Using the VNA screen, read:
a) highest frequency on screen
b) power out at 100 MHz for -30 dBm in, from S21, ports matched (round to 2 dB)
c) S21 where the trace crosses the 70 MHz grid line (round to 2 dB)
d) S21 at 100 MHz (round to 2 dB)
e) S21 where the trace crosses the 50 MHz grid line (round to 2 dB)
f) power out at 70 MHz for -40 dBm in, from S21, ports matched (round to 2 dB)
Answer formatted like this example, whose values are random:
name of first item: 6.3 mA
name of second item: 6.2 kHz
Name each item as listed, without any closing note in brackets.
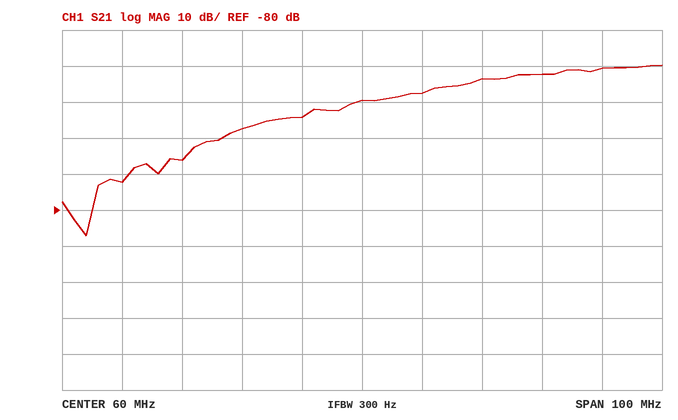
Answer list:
highest frequency on screen: 110 MHz
power out at 100 MHz for -30 dBm in, from S21, ports matched: -70 dBm
S21 where the trace crosses the 70 MHz grid line: -48 dB
S21 at 100 MHz: -40 dB
S21 where the trace crosses the 50 MHz grid line: -54 dB
power out at 70 MHz for -40 dBm in, from S21, ports matched: -88 dBm
